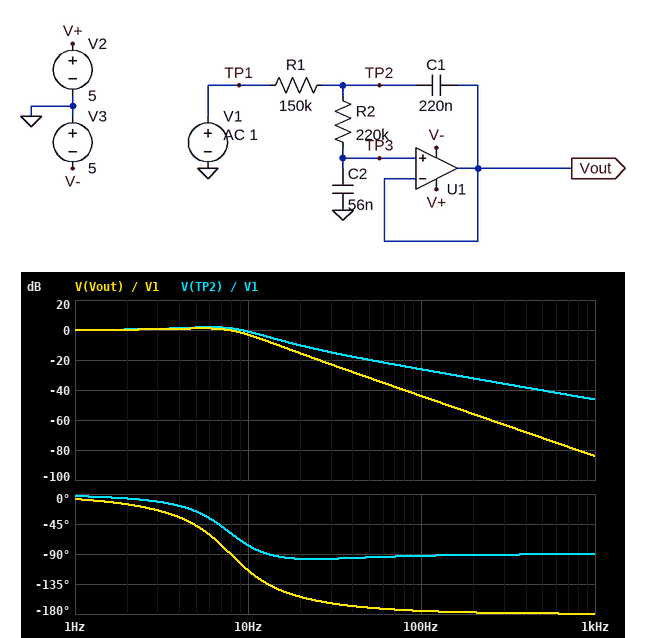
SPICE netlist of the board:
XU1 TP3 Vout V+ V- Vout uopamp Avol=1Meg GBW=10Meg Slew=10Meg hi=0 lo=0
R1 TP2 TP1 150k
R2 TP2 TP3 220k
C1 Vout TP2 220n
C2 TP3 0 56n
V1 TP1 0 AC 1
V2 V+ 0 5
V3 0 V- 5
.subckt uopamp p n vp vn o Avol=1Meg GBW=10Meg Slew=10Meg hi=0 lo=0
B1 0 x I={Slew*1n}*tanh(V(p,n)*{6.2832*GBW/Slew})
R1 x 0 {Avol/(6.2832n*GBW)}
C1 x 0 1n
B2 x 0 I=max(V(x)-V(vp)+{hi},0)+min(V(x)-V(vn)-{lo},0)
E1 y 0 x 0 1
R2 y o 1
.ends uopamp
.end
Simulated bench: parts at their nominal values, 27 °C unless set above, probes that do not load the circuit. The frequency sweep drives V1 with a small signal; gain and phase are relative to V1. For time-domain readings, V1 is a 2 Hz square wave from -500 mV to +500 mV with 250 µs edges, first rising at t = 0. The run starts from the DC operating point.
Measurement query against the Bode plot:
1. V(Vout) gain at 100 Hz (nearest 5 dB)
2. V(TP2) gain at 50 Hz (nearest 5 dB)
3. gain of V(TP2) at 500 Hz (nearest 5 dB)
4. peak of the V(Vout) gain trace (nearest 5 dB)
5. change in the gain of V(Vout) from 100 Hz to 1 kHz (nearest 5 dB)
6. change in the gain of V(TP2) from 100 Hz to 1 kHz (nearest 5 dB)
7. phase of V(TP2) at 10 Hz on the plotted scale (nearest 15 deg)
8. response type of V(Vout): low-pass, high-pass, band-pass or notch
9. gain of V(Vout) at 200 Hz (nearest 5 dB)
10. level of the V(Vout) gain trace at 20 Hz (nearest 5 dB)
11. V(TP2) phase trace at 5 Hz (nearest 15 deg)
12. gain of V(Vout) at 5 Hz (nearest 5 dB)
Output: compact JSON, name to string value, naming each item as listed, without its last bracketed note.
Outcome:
{"V(Vout) gain at 100 Hz": "-45 dB", "V(TP2) gain at 50 Hz": "-20 dB", "gain of V(TP2) at 500 Hz": "-40 dB", "peak of the V(Vout) gain trace": "0 dB", "change in the gain of V(Vout) from 100 Hz to 1 kHz": "-40 dB", "change in the gain of V(TP2) from 100 Hz to 1 kHz": "-20 dB", "phase of V(TP2) at 10 Hz on the plotted scale": "-75 deg", "response type of V(Vout): low-pass, high-pass, band-pass or notch": "low-pass", "gain of V(Vout) at 200 Hz": "-55 dB", "level of the V(Vout) gain trace at 20 Hz": "-15 dB", "V(TP2) phase trace at 5 Hz": "-30 deg", "gain of V(Vout) at 5 Hz": "0 dB"}
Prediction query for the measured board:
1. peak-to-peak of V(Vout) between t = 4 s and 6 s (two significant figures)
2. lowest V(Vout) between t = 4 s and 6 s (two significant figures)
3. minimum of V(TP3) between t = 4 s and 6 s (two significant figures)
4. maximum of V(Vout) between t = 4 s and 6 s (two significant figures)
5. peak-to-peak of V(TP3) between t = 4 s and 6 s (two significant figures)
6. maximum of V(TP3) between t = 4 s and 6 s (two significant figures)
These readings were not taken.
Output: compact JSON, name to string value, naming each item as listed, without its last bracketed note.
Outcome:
{"peak-to-peak of V(Vout) between t = 4 s and 6 s": "1.3 V", "lowest V(Vout) between t = 4 s and 6 s": "-650 mV", "minimum of V(TP3) between t = 4 s and 6 s": "-650 mV", "maximum of V(Vout) between t = 4 s and 6 s": "650 mV", "peak-to-peak of V(TP3) between t = 4 s and 6 s": "1.3 V", "maximum of V(TP3) between t = 4 s and 6 s": "650 mV"}
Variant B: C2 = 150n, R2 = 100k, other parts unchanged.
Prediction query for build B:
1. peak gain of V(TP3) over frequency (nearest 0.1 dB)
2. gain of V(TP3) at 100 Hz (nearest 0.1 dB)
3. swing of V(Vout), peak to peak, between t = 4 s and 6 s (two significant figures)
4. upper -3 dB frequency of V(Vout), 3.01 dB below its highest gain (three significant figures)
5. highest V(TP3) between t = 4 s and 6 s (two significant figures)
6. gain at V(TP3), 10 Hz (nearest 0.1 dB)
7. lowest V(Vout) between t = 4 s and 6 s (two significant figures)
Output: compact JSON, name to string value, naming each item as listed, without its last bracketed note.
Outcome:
{"peak gain of V(TP3) over frequency": "0 dB", "gain of V(TP3) at 100 Hz": "-45.8 dB", "swing of V(Vout), peak to peak, between t = 4 s and 6 s": "1.0 V", "upper -3 dB frequency of V(Vout), 3.01 dB below its highest gain": "5.83 Hz", "highest V(TP3) between t = 4 s and 6 s": "510 mV", "gain at V(TP3), 10 Hz": "-8.1 dB", "lowest V(Vout) between t = 4 s and 6 s": "-510 mV"}
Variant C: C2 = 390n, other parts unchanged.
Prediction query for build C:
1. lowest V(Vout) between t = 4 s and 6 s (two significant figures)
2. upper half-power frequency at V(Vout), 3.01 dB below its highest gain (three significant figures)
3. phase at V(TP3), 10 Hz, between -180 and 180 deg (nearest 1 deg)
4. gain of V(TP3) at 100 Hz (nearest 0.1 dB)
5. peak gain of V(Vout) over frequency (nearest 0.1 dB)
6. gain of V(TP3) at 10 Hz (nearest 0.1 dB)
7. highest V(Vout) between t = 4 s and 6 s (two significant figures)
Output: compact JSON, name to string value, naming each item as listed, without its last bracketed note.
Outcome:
{"lowest V(Vout) between t = 4 s and 6 s": "-360 mV", "upper half-power frequency at V(Vout), 3.01 dB below its highest gain": "1.27 Hz", "phase at V(TP3), 10 Hz, between -180 and 180 deg": "-138 deg", "gain of V(TP3) at 100 Hz": "-61.0 dB", "peak gain of V(Vout) over frequency": "0 dB", "gain of V(TP3) at 10 Hz": "-22.7 dB", "highest V(Vout) between t = 4 s and 6 s": "360 mV"}
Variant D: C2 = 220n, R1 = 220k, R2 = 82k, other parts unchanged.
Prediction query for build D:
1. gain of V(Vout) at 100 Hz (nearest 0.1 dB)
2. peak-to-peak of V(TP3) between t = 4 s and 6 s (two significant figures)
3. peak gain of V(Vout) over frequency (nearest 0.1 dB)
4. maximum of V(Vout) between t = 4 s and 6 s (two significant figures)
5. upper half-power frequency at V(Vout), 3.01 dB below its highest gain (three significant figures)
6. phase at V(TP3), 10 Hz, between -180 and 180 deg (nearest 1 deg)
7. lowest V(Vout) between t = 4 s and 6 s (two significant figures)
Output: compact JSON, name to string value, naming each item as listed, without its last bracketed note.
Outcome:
{"gain of V(Vout) at 100 Hz": "-50.8 dB", "peak-to-peak of V(TP3) between t = 4 s and 6 s": "980 mV", "peak gain of V(Vout) over frequency": "0 dB", "maximum of V(Vout) between t = 4 s and 6 s": "490 mV", "upper half-power frequency at V(Vout), 3.01 dB below its highest gain": "2.94 Hz", "phase at V(TP3), 10 Hz, between -180 and 180 deg": "-120 deg", "lowest V(Vout) between t = 4 s and 6 s": "-490 mV"}
